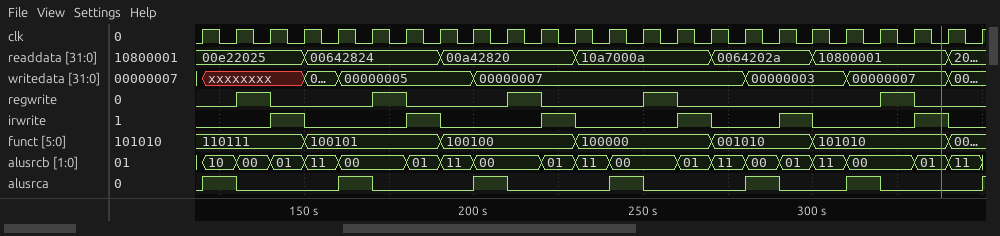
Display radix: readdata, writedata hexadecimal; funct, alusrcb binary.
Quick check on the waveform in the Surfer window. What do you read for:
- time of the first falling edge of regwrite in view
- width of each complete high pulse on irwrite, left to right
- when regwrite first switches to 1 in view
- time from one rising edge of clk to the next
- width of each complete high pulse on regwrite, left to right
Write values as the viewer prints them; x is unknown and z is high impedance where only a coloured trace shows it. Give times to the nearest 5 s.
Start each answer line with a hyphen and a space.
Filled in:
- 140 s
- 10 s, 10 s, 10 s, 10 s, 10 s, 10 s
- 130 s
- 10 s
- 10 s, 10 s, 10 s, 10 s, 10 s
